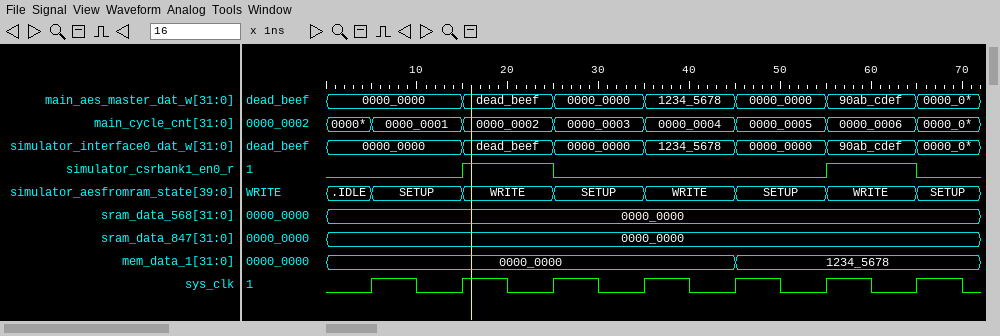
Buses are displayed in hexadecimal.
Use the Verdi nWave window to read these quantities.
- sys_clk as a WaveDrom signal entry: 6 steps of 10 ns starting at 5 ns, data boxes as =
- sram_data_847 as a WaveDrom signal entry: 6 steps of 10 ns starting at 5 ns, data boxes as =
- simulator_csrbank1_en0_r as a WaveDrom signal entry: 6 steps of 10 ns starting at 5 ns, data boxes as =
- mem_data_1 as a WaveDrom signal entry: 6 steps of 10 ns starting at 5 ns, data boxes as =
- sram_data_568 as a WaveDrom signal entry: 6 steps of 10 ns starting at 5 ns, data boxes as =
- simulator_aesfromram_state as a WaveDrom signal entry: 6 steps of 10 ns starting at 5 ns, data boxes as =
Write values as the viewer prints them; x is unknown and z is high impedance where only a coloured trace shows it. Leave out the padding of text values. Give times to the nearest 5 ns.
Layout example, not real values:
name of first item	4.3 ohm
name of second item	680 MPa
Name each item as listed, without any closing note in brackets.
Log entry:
sys_clk as a WaveDrom signal entry: 6 steps of 10 ns starting at 5 ns, data boxes as =	{name: 'sys_clk', wave: 'p.....'}
sram_data_847 as a WaveDrom signal entry: 6 steps of 10 ns starting at 5 ns, data boxes as =	{name: 'sram_data_847', wave: '=.....', data: '0000_0000'}
simulator_csrbank1_en0_r as a WaveDrom signal entry: 6 steps of 10 ns starting at 5 ns, data boxes as =	{name: 'simulator_csrbank1_en0_r', wave: '010..1'}
mem_data_1 as a WaveDrom signal entry: 6 steps of 10 ns starting at 5 ns, data boxes as =	{name: 'mem_data_1', wave: '=...=.', data: '0000_0000 1234_5678'}
sram_data_568 as a WaveDrom signal entry: 6 steps of 10 ns starting at 5 ns, data boxes as =	{name: 'sram_data_568', wave: '=.....', data: '0000_0000'}
simulator_aesfromram_state as a WaveDrom signal entry: 6 steps of 10 ns starting at 5 ns, data boxes as =	{name: 'simulator_aesfromram_state', wave: '======', data: 'SETUP WRITE SETUP WRITE SETUP WRITE'}
